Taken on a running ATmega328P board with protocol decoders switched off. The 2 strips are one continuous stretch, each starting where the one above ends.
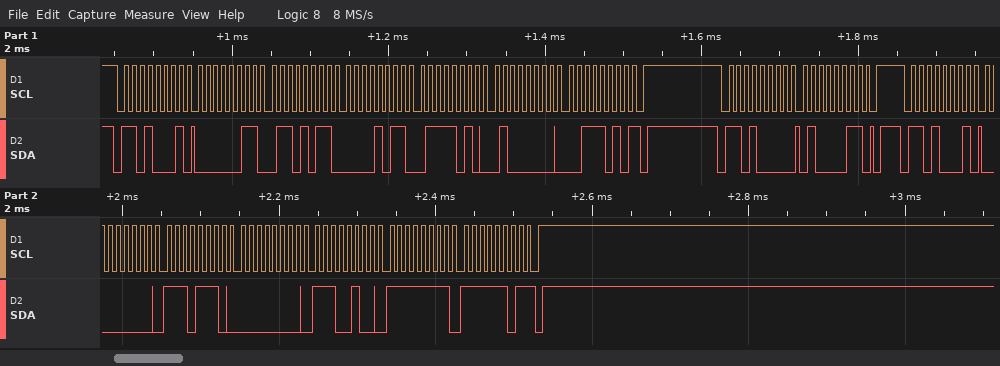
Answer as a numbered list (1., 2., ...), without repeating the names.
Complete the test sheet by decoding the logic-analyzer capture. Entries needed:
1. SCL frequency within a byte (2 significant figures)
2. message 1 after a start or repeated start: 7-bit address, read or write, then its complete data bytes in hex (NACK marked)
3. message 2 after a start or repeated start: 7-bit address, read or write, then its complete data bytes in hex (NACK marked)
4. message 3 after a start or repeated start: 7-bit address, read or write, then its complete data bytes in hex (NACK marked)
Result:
1. 100 kHz
2. 0x68 read: 03 6B 0B 7A 40 3A NACK
3. 0x68 write: 43
4. 0x68 read: 00 EE 00 E4 FF FD NACK
